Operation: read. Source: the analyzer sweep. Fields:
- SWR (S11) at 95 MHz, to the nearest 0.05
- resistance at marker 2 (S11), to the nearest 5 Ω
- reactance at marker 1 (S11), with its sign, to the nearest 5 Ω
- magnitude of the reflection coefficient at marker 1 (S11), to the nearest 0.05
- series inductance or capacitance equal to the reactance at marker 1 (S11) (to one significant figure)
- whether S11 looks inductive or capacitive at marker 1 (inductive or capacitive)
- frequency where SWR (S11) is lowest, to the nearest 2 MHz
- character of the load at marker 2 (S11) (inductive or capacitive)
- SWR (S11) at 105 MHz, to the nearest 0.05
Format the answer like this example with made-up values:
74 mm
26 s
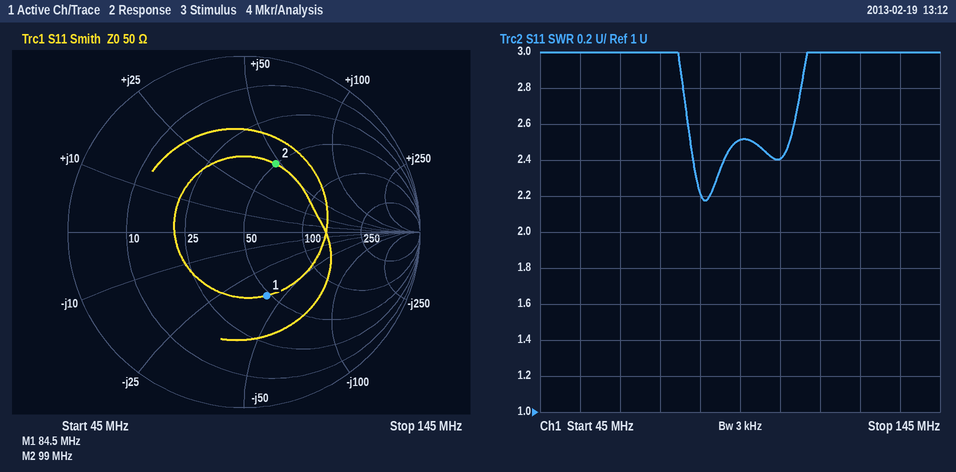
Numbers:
2.50
50 Ω
-40 Ω
0.40
50 pF
capacitive
86 MHz
inductive
2.40
